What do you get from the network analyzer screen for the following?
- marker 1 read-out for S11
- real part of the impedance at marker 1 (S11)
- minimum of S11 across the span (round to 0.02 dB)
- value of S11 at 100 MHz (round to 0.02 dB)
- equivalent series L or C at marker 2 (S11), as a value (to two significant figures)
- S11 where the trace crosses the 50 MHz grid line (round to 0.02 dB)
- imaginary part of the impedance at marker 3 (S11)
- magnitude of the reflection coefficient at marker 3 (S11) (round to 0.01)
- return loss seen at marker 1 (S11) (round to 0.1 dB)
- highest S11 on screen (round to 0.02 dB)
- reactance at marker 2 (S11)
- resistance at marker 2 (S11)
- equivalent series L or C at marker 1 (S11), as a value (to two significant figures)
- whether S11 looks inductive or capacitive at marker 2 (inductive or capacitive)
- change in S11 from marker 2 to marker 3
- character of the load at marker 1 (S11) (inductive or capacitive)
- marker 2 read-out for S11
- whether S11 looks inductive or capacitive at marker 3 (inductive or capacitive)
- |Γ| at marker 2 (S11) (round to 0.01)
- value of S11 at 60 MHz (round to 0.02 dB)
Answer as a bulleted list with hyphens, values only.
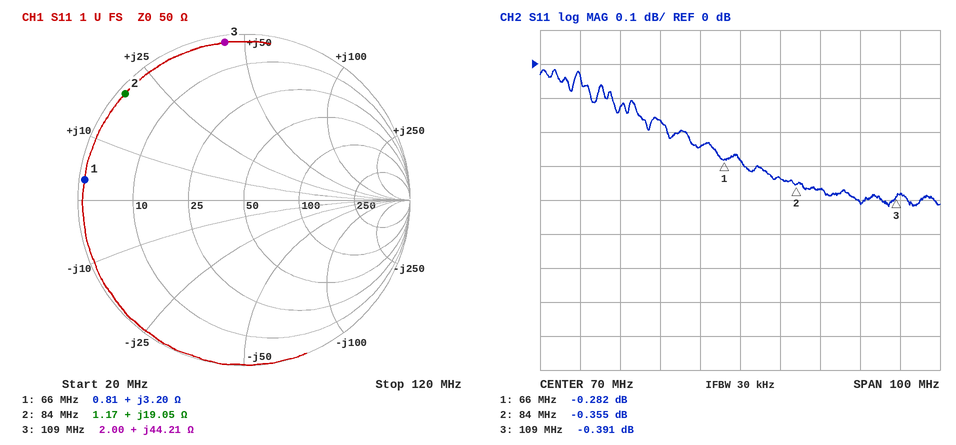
- -0.282 dB
- 0.81 Ω
- -0.42 dB
- -0.40 dB
- 36 nH
- -0.16 dB
- +44.21 Ω
- 0.96
- 0.3 dB
- -0.02 dB
- +19.05 Ω
- 1.17 Ω
- 7.7 nH
- inductive
- -0.036 dB
- inductive
- -0.355 dB
- inductive
- 0.96
- -0.24 dB
